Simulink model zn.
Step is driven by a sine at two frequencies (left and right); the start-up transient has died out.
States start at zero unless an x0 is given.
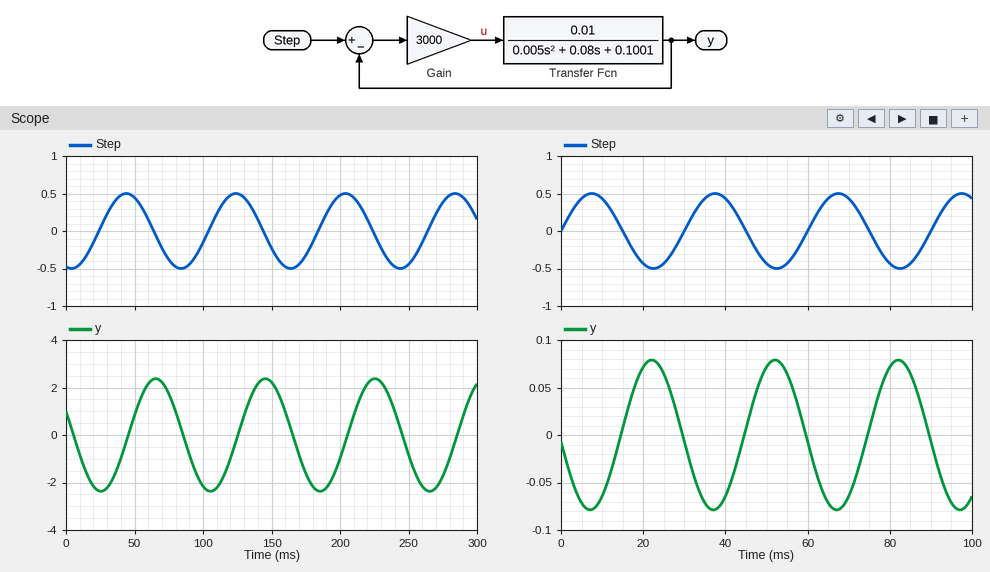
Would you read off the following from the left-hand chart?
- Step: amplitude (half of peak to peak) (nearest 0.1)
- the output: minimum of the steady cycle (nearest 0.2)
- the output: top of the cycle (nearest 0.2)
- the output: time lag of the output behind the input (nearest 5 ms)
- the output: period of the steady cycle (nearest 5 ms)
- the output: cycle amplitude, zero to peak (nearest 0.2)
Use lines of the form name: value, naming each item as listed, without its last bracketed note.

Step: amplitude (half of peak to peak): 0.5
the output: minimum of the steady cycle: -2.4
the output: top of the cycle: 2.4
the output: time lag of the output behind the input: 20 ms
the output: period of the steady cycle: 80 ms
the output: cycle amplitude, zero to peak: 2.4
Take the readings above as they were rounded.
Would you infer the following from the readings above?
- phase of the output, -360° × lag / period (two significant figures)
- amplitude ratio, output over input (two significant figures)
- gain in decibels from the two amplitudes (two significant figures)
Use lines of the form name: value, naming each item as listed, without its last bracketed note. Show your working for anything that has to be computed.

phase of the output, -360° × lag / period: -360 × 20 / 80 = -90°
amplitude ratio, output over input: 2.4 / 0.5 = 4.8
gain in decibels from the two amplitudes: 20 log10(2.4 / 0.5) = 14 dB
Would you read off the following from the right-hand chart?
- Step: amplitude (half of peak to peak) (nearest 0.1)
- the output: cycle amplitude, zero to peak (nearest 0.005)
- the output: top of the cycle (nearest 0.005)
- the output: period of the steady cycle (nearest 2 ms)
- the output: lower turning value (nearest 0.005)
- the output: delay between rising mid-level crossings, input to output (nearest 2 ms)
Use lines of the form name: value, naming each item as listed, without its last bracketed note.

Step: amplitude (half of peak to peak): 0.5
the output: cycle amplitude, zero to peak: 0.080
the output: top of the cycle: 0.080
the output: period of the steady cycle: 30 ms
the output: lower turning value: -0.080
the output: delay between rising mid-level crossings, input to output: 14 ms
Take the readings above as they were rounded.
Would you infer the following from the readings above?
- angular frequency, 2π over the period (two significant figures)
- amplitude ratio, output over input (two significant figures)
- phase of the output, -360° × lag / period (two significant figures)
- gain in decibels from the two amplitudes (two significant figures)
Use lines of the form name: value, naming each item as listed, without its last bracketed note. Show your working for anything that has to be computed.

angular frequency, 2π over the period: 2π / 30 = 0.21 rad/ms
amplitude ratio, output over input: 0.08 / 0.5 = 0.16
phase of the output, -360° × lag / period: -360 × 14 / 30 = -170°
gain in decibels from the two amplitudes: 20 log10(0.08 / 0.5) = -16 dB
